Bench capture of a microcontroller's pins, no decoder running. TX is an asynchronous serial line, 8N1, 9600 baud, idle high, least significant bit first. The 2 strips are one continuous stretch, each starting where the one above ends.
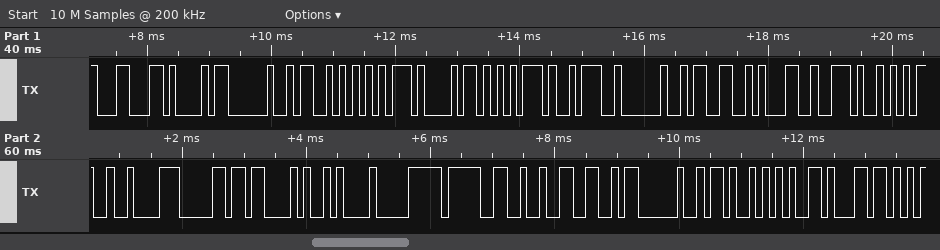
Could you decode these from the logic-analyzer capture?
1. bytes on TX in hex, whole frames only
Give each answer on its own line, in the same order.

8C A1 20 53 75 68 75 3A 20 33 31 2E 35 C2 B0 43 0A F0 9F 92 A6 20 4B 65 6C
